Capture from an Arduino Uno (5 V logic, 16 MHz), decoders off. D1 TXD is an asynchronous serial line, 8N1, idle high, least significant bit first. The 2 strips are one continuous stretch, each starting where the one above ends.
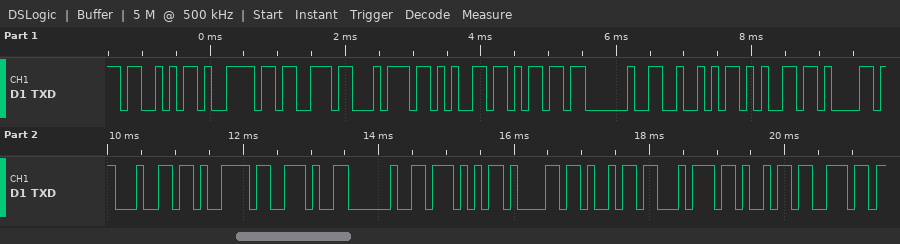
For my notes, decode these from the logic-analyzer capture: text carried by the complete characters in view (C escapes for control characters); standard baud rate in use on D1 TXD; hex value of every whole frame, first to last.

"System Ready. Waitin"
9600 baud
53 79 73 74 65 6D 20 52 65 61 64 79 2E 20 57 61 69 74 69 6E
